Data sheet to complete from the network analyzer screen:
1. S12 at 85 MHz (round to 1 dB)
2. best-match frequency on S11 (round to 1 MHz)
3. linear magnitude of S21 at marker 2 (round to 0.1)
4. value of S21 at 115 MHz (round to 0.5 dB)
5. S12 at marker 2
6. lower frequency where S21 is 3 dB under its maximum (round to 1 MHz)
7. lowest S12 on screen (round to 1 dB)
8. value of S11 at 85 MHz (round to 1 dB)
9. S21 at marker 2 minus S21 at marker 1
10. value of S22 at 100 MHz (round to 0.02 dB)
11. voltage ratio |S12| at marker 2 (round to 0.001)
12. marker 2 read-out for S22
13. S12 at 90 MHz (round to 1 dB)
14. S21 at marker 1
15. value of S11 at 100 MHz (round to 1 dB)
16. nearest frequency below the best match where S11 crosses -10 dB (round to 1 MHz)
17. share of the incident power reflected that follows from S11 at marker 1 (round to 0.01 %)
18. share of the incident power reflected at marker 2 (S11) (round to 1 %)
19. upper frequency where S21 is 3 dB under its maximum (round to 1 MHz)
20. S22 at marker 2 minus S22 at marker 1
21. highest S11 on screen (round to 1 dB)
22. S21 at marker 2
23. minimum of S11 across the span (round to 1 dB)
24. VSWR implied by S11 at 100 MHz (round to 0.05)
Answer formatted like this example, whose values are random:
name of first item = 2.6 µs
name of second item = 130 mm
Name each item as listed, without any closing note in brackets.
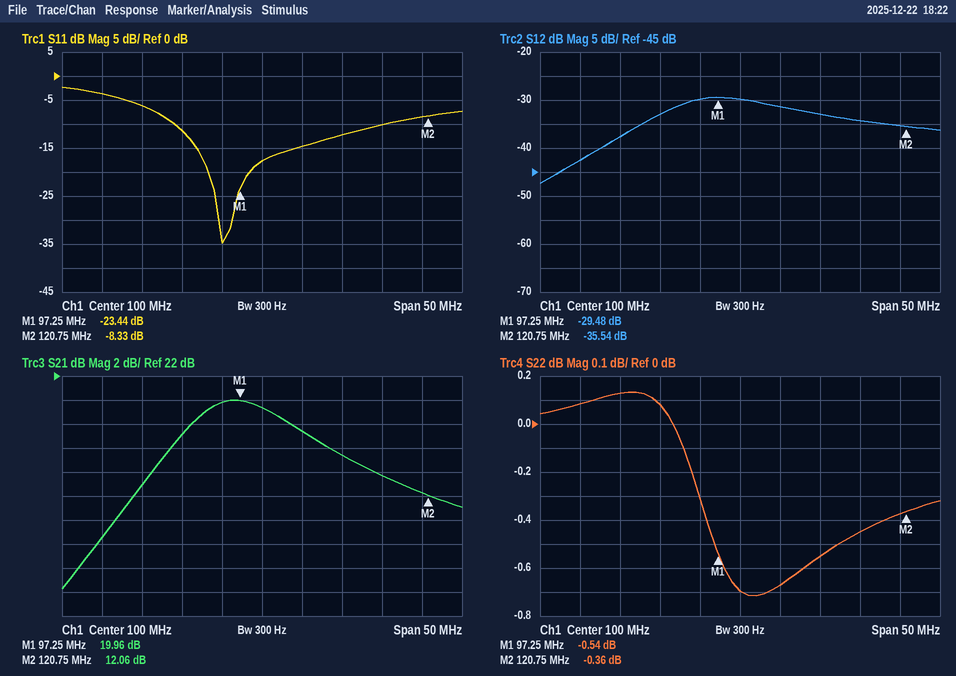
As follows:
S12 at 85 MHz = -38 dB
best-match frequency on S11 = 95 MHz
linear magnitude of S21 at marker 2 = 4.0
value of S21 at 115 MHz = 13.5 dB
S12 at marker 2 = -35.54 dB
lower frequency where S21 is 3 dB under its maximum = 90 MHz
lowest S12 on screen = -47 dB
value of S11 at 85 MHz = -6 dB
S21 at marker 2 minus S21 at marker 1 = -7.90 dB
value of S22 at 100 MHz = -0.70 dB
voltage ratio |S12| at marker 2 = 0.017
marker 2 read-out for S22 = -0.36 dB
S12 at 90 MHz = -33 dB
S21 at marker 1 = 19.96 dB
value of S11 at 100 MHz = -18 dB
nearest frequency below the best match where S11 crosses -10 dB = 89 MHz
share of the incident power reflected that follows from S11 at marker 1 = 0.45 %
share of the incident power reflected at marker 2 (S11) = 15 %
upper frequency where S21 is 3 dB under its maximum = 106 MHz
S22 at marker 2 minus S22 at marker 1 = 0.18 dB
highest S11 on screen = -2 dB
S21 at marker 2 = 12.06 dB
minimum of S11 across the span = -35 dB
VSWR implied by S11 at 100 MHz = 1.30
